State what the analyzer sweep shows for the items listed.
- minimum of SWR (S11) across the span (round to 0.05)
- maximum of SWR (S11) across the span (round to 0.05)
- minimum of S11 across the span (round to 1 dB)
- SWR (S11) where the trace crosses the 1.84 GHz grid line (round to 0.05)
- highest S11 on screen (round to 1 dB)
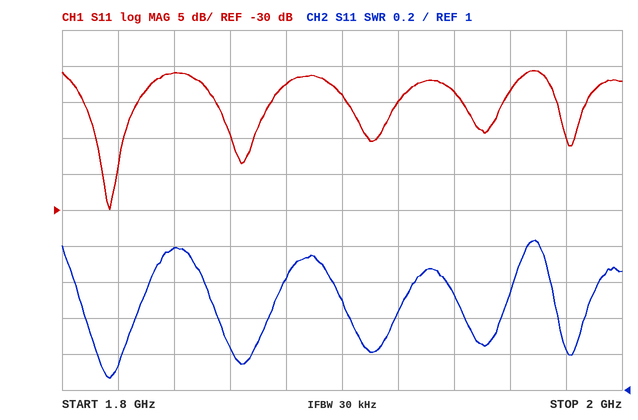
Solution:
1.05
1.85
-30 dB
1.80
-11 dB
